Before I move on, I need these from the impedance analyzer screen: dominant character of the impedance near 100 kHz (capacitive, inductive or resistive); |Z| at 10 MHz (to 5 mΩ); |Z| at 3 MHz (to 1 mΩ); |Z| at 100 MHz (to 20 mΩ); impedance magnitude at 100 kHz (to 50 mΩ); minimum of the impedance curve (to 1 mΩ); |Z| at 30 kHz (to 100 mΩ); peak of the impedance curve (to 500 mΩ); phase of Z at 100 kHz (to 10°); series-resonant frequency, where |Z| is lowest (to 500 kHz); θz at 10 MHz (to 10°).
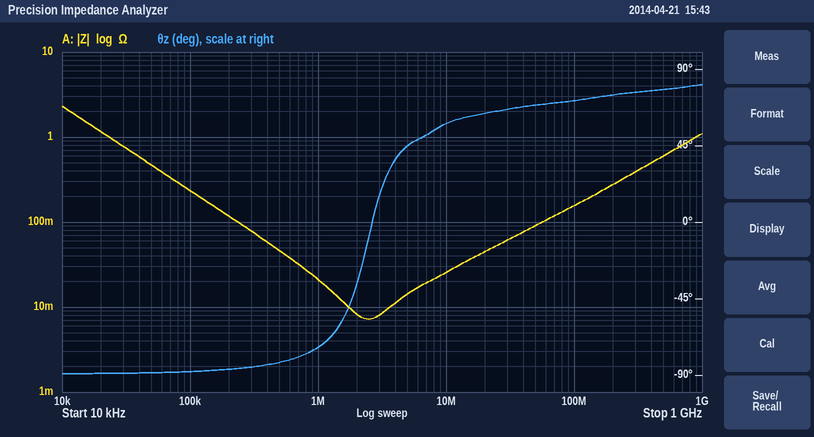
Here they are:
capacitive
25 mΩ
8 mΩ
160 mΩ
250 mΩ
7 mΩ
800 mΩ
2.5 Ω
-90°
2.5 MHz
60°
